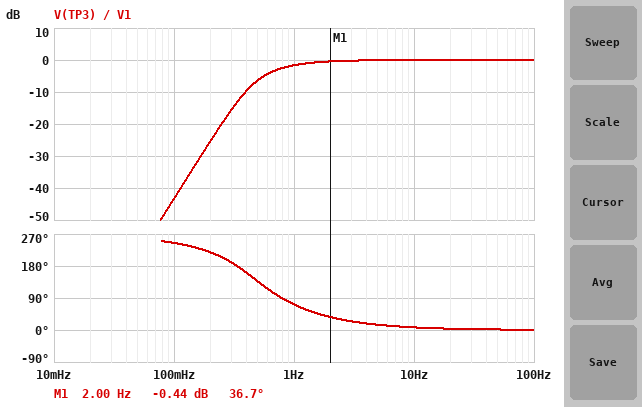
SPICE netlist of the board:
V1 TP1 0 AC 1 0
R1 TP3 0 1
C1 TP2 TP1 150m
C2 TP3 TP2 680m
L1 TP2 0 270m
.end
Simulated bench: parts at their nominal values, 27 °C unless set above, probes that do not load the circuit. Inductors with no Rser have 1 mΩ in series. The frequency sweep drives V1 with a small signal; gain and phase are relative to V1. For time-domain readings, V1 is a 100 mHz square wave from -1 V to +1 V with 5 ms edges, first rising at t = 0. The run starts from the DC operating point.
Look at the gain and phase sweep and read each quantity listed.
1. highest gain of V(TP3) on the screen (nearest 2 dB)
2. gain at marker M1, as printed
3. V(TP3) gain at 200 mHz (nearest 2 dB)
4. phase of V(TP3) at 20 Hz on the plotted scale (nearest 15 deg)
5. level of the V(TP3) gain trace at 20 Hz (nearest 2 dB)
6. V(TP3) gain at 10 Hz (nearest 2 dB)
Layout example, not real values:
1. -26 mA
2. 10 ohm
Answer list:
1. 0 dB
2. -0.44 dB
3. -26 dB
4. 0 deg
5. 0 dB
6. 0 dB
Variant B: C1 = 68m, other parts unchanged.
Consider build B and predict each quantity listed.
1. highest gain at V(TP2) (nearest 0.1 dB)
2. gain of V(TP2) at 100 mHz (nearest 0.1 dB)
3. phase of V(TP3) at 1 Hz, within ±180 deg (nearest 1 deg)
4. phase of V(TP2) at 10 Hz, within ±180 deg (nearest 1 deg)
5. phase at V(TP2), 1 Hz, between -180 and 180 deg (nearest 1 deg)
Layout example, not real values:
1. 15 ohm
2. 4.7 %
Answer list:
1. 0 dB
2. -42.2 dB
3. 100 deg
4. 13 deg
5. 86 deg
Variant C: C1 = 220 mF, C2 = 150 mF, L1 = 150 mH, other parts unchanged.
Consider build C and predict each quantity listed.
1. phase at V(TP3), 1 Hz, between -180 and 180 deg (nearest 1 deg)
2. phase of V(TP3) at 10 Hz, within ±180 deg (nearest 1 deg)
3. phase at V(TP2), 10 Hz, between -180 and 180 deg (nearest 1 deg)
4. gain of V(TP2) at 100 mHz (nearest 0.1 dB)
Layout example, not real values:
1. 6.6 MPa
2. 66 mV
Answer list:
1. 77 deg
2. 10 deg
3. 4 deg
4. -37.5 dB
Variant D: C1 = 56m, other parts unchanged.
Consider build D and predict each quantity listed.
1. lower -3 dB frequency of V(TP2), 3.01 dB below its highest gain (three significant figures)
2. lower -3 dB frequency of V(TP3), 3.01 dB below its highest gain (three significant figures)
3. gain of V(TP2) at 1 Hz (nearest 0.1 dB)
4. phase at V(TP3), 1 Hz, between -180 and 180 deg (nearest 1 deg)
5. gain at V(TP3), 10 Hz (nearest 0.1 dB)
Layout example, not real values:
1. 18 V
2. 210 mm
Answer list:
1. 2.46 Hz
2. 2.49 Hz
3. -8.6 dB
4. 104 deg
5. -0.3 dB
